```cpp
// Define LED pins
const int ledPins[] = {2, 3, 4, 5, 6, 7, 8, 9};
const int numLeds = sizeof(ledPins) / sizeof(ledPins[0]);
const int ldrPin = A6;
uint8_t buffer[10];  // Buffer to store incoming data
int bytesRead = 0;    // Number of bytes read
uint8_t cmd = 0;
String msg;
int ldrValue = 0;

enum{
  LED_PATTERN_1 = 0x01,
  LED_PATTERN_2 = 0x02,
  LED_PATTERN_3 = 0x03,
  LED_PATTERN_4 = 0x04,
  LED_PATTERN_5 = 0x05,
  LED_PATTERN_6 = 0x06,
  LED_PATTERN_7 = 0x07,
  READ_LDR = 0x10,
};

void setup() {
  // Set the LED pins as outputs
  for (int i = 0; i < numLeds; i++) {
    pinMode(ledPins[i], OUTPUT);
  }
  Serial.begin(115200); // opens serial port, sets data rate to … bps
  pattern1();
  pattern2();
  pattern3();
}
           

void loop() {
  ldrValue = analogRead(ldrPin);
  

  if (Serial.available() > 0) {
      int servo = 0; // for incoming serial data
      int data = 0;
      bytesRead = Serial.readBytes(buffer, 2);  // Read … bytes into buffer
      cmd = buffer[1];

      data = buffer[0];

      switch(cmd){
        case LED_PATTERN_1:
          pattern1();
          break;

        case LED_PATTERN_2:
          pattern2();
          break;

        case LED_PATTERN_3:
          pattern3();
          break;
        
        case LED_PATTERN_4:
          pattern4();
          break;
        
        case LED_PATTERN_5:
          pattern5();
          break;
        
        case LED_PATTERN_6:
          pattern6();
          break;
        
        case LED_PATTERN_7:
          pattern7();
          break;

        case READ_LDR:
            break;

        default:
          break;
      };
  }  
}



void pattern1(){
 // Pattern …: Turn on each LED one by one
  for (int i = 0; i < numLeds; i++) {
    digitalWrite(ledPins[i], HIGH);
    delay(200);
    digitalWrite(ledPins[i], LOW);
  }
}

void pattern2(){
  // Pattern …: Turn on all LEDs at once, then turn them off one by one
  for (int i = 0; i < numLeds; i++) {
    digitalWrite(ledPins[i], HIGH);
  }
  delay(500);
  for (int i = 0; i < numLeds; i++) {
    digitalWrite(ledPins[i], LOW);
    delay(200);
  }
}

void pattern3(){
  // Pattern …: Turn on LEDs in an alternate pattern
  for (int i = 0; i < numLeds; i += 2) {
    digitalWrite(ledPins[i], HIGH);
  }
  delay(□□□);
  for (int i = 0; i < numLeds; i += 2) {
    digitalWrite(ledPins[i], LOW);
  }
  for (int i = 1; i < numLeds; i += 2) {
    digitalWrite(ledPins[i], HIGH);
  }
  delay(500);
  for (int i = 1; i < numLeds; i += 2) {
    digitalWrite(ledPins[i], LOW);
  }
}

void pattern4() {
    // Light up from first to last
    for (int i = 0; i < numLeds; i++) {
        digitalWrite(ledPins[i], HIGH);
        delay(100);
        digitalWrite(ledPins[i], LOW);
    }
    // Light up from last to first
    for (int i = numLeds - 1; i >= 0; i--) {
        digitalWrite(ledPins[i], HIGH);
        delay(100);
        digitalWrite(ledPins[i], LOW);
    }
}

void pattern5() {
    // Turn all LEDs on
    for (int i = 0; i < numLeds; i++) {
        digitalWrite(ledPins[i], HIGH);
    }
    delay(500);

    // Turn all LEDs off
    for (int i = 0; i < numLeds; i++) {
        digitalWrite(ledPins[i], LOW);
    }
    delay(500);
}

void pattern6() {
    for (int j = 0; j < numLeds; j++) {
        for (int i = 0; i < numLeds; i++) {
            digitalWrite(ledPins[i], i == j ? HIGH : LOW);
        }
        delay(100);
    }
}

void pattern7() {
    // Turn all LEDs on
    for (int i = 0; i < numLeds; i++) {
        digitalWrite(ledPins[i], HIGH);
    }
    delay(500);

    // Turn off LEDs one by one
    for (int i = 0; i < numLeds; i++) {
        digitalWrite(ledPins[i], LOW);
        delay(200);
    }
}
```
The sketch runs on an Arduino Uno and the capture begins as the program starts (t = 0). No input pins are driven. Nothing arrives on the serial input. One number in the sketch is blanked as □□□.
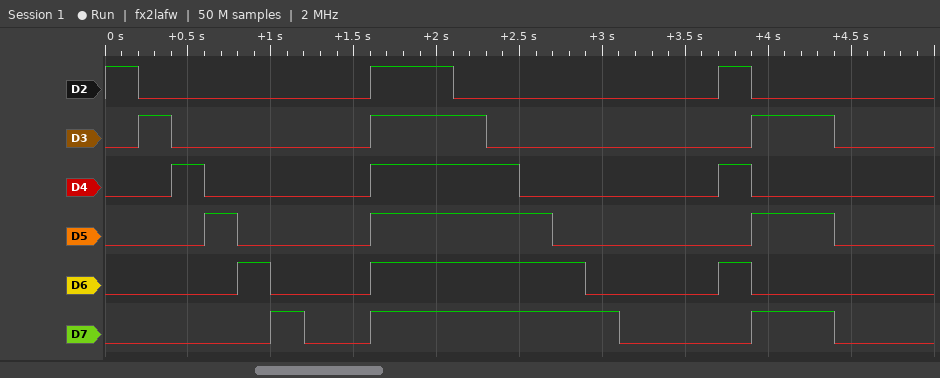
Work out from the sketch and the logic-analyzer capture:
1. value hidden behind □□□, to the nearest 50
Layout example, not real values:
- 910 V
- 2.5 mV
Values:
- 200
